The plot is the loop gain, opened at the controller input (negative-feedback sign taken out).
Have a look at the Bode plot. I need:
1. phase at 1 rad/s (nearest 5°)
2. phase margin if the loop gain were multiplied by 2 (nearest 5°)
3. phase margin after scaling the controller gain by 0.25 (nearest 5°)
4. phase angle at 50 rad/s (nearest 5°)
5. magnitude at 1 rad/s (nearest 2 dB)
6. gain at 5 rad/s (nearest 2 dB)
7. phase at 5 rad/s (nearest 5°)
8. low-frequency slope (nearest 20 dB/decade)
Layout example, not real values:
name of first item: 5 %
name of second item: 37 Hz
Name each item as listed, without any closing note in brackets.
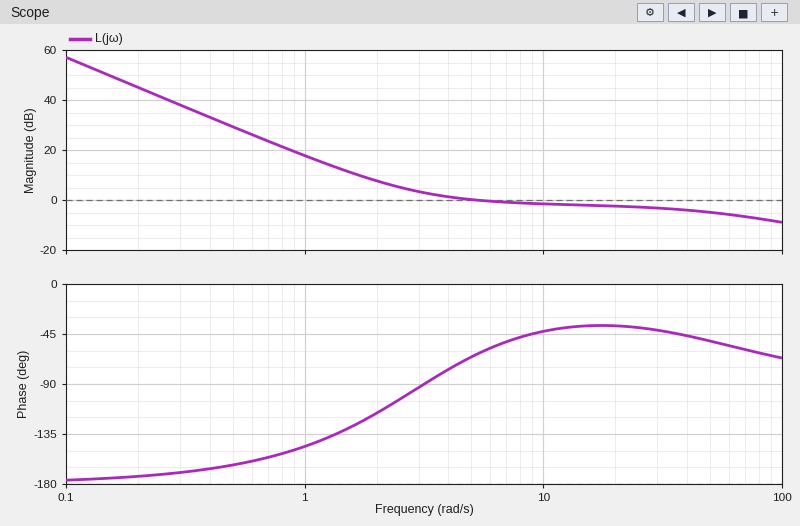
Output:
phase at 1 rad/s: -145°
phase margin if the loop gain were multiplied by 2: 125°
phase margin after scaling the controller gain by 0.25: 50°
phase angle at 50 rad/s: -50°
magnitude at 1 rad/s: 18 dB
gain at 5 rad/s: 0 dB
phase at 5 rad/s: -65°
low-frequency slope: -40 dB/decade
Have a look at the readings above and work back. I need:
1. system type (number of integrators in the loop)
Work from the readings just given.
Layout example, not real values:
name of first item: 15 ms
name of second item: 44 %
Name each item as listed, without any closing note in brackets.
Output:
system type: 2
